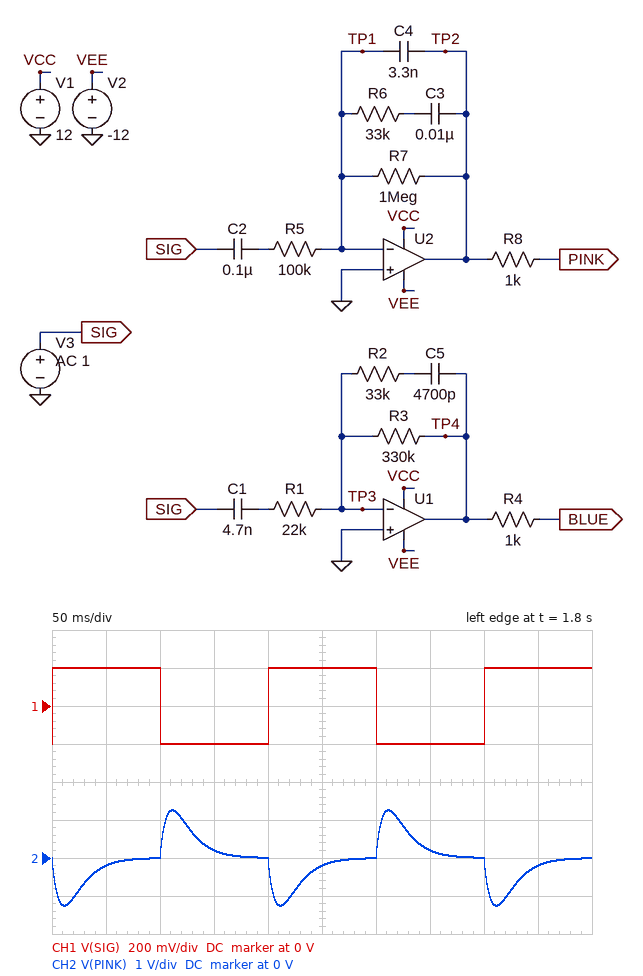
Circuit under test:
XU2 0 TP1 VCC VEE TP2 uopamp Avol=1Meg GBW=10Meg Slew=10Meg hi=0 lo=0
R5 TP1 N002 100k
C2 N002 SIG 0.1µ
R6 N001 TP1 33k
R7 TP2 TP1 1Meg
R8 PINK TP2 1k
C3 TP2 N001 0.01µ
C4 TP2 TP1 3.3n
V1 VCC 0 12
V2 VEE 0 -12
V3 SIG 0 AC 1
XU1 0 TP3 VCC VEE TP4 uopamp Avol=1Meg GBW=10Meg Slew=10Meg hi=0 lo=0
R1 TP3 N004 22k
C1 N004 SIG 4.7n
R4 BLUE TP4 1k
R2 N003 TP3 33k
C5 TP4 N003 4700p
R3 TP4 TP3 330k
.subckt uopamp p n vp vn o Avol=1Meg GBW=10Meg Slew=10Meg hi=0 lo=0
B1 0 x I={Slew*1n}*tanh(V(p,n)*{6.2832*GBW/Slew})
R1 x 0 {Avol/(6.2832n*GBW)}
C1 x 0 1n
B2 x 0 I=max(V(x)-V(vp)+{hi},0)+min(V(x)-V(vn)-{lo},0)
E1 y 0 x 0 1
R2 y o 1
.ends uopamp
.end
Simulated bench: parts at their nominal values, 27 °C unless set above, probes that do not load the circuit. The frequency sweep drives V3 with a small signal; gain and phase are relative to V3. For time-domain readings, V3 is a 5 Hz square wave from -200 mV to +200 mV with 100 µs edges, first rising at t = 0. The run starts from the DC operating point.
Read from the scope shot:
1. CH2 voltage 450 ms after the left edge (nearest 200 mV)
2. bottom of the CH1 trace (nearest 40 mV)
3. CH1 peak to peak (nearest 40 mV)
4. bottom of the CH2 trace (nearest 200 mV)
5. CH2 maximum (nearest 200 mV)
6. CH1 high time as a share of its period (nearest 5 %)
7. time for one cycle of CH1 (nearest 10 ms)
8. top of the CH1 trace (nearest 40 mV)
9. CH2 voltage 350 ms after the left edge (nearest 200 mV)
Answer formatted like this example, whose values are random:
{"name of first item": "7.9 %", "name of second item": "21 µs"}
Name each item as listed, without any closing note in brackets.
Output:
{"CH2 voltage 450 ms after the left edge": "-200 mV", "bottom of the CH1 trace": "-200 mV", "CH1 peak to peak": "400 mV", "bottom of the CH2 trace": "-1.2 V", "CH2 maximum": "1.2 V", "CH1 high time as a share of its period": "50 %", "time for one cycle of CH1": "200 ms", "top of the CH1 trace": "200 mV", "CH2 voltage 350 ms after the left edge": "200 mV"}
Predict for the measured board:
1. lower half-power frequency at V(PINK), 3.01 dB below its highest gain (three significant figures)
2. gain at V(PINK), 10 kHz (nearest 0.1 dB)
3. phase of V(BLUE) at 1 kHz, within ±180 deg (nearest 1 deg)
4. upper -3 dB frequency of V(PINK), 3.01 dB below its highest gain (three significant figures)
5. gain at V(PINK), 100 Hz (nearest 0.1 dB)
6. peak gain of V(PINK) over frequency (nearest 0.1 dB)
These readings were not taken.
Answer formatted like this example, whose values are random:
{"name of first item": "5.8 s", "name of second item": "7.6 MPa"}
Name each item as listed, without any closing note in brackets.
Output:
{"lower half-power frequency at V(PINK), 3.01 dB below its highest gain": "5.62 Hz", "gain at V(PINK), 10 kHz": "-26.5 dB", "phase of V(BLUE) at 1 kHz, within ±180 deg": "-163 deg", "upper -3 dB frequency of V(PINK), 3.01 dB below its highest gain": "33.4 Hz", "gain at V(PINK), 100 Hz": "1.4 dB", "peak gain of V(PINK) over frequency": "12.6 dB"}
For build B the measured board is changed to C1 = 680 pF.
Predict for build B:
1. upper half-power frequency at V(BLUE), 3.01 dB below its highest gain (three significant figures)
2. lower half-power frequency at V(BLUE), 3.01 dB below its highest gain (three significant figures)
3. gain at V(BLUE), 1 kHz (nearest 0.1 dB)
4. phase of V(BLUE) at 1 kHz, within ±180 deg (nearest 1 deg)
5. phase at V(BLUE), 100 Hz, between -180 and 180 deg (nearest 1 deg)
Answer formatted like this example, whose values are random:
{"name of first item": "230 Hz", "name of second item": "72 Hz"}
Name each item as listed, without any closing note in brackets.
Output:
{"upper half-power frequency at V(BLUE), 3.01 dB below its highest gain": "4.25 MHz", "lower half-power frequency at V(BLUE), 3.01 dB below its highest gain": "10.5 kHz", "gain at V(BLUE), 1 kHz": "-14.8 dB", "phase of V(BLUE) at 1 kHz, within ±180 deg": "-136 deg", "phase at V(BLUE), 100 Hz, between -180 and 180 deg": "-132 deg"}
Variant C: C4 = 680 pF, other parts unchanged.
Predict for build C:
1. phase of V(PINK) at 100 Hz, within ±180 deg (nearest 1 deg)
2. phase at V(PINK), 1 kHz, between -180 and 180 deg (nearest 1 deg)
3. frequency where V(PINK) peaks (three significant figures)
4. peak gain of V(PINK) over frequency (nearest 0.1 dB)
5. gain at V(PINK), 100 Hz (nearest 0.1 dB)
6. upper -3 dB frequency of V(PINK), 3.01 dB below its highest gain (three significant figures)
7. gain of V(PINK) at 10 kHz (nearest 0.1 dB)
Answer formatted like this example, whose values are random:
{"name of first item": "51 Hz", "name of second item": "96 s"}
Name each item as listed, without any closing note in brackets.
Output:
{"phase of V(PINK) at 100 Hz, within ±180 deg": "118 deg", "phase at V(PINK), 1 kHz, between -180 and 180 deg": "149 deg", "frequency where V(PINK) peaks": "15.2 Hz", "peak gain of V(PINK) over frequency": "13.6 dB", "gain at V(PINK), 100 Hz": "3.2 dB", "upper -3 dB frequency of V(PINK), 3.01 dB below its highest gain": "36.8 Hz", "gain of V(PINK) at 10 kHz": "-14.7 dB"}
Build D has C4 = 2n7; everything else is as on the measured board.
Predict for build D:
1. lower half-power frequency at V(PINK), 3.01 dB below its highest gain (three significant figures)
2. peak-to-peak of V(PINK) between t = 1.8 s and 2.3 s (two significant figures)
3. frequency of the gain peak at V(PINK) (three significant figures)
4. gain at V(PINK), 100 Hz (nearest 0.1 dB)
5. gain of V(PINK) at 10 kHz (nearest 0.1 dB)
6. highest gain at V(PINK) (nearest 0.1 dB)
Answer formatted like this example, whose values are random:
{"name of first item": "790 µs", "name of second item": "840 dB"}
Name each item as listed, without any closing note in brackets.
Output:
{"lower half-power frequency at V(PINK), 3.01 dB below its highest gain": "5.76 Hz", "peak-to-peak of V(PINK) between t = 1.8 s and 2.3 s": "2.6 V", "frequency of the gain peak at V(PINK)": "14.0 Hz", "gain at V(PINK), 100 Hz": "1.8 dB", "gain of V(PINK) at 10 kHz": "-24.8 dB", "highest gain at V(PINK)": "12.8 dB"}
